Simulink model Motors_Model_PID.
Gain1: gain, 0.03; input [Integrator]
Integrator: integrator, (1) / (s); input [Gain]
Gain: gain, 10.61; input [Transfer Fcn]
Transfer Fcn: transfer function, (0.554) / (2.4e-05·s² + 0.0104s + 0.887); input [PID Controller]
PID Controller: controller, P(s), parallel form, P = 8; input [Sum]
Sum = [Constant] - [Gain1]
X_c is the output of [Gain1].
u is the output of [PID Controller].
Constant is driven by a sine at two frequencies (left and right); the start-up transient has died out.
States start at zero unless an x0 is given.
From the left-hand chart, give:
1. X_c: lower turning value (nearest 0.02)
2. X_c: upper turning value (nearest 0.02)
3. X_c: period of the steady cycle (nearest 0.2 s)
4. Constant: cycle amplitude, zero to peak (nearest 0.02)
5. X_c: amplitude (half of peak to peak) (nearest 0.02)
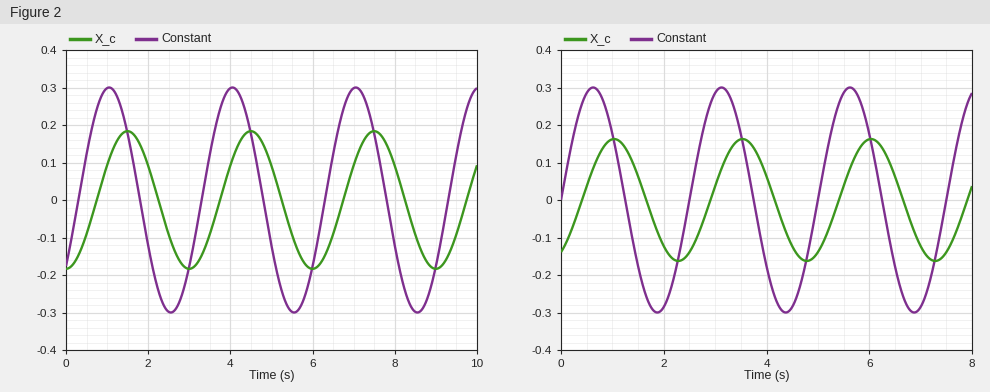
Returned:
-0.18
0.18
3.0 s
0.30
0.18
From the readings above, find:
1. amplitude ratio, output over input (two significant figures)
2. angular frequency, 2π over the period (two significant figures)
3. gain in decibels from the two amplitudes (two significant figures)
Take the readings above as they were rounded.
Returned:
0.60
2.1 rad/s
-4.4 dB
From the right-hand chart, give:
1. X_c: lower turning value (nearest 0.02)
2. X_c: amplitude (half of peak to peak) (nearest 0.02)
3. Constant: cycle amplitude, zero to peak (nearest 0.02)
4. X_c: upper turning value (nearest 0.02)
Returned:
-0.16
0.16
0.30
0.16
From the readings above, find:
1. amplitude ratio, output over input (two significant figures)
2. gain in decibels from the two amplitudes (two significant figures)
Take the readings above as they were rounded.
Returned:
0.53
-5.5 dB
